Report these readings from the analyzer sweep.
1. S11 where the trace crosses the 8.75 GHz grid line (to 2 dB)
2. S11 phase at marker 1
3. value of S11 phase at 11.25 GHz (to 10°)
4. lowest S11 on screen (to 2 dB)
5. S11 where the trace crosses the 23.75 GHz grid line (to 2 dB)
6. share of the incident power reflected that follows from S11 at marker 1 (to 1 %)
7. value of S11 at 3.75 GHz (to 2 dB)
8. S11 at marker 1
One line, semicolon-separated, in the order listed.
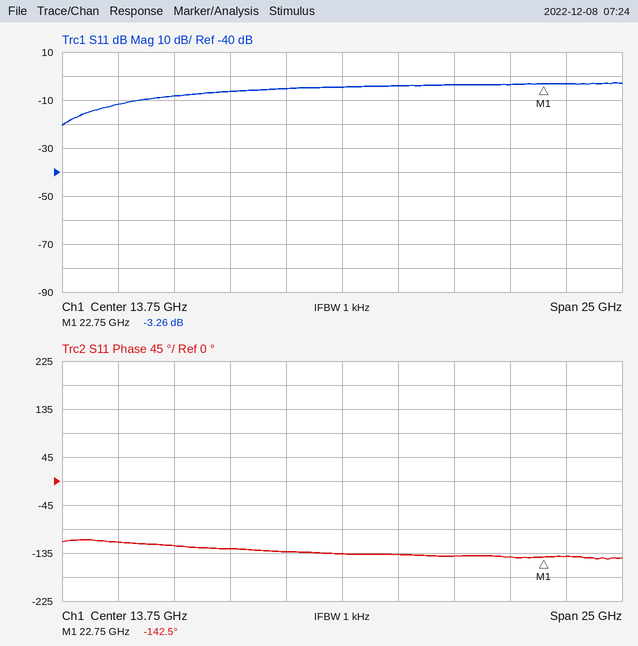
-6 dB; -142.5°; -130°; -20 dB; -4 dB; 47 %; -12 dB; -3.26 dB
